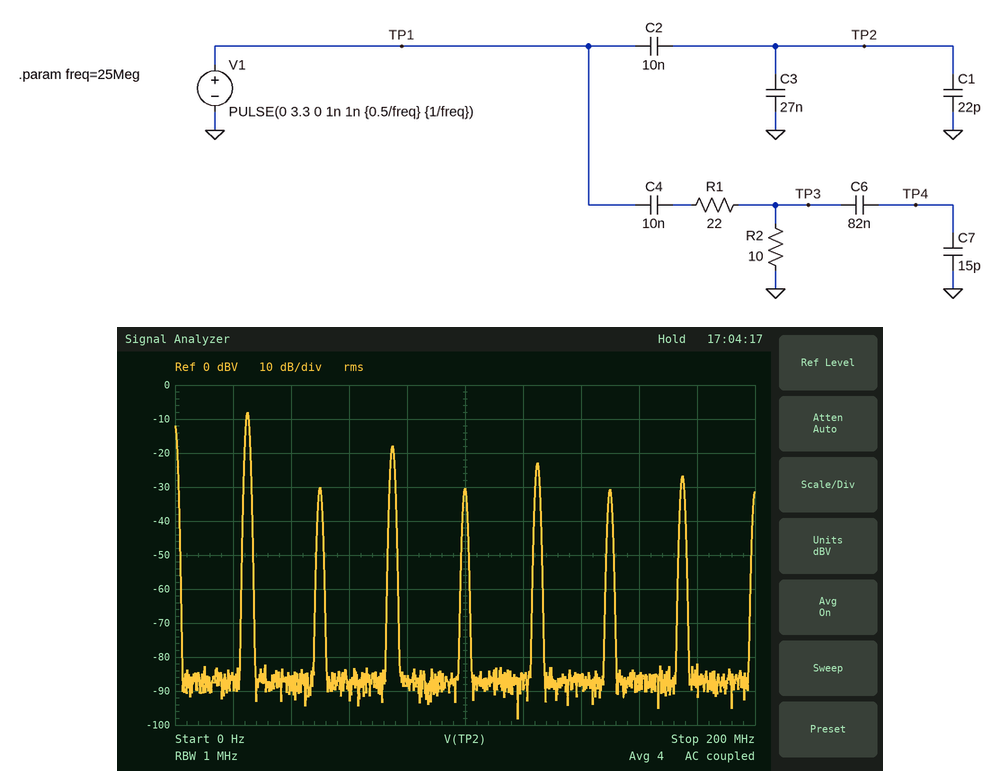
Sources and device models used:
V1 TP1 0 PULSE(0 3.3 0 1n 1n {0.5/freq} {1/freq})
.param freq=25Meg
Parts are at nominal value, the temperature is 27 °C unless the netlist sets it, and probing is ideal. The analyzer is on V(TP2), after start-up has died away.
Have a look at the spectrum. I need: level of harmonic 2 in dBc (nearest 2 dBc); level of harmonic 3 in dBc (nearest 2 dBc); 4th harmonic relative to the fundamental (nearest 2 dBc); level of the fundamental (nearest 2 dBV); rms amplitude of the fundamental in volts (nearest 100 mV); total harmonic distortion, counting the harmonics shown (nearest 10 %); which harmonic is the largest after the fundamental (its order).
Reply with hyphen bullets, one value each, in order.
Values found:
- -22 dBc
- -10 dBc
- -22 dBc
- -8 dBV
- 400 mV
- 40 %
- 3
